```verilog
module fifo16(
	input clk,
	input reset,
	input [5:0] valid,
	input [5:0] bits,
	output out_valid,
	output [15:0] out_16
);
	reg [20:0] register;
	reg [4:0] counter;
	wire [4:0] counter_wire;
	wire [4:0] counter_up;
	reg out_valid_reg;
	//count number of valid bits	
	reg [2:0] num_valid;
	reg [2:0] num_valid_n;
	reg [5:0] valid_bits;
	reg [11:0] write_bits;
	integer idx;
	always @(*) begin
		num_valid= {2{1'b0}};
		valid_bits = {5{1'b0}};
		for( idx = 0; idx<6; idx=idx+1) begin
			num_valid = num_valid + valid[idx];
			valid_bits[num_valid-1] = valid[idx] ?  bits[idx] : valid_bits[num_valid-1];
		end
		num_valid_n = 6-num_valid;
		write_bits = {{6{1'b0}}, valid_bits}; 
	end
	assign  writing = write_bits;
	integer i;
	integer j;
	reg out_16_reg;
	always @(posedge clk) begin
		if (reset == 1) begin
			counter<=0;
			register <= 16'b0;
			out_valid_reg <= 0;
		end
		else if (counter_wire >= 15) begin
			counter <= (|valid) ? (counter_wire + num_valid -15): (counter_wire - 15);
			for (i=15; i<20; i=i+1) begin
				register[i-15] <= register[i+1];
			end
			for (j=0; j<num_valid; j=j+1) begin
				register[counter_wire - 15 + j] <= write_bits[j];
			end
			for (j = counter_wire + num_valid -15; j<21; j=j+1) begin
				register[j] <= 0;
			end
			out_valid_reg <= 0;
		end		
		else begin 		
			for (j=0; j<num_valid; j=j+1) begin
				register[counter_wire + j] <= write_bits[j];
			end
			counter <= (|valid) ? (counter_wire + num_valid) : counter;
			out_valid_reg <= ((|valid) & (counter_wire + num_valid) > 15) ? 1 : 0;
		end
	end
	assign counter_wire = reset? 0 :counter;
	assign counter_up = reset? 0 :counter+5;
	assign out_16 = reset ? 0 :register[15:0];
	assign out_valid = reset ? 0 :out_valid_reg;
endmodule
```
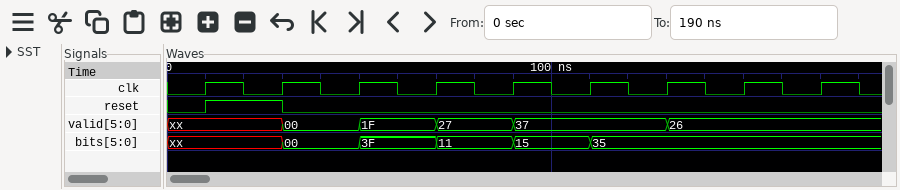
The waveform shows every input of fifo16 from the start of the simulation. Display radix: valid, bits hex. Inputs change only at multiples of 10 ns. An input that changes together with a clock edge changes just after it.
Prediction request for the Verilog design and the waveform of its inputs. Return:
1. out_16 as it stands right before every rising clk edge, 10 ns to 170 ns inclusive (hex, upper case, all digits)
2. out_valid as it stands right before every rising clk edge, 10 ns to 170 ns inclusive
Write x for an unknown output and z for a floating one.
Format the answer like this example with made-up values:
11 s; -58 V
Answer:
x, 0000, 0000, 0000, 001F, 003F, 1A3F, 5A3F, 0067; x 0 0 0 0 0 0 1 0
